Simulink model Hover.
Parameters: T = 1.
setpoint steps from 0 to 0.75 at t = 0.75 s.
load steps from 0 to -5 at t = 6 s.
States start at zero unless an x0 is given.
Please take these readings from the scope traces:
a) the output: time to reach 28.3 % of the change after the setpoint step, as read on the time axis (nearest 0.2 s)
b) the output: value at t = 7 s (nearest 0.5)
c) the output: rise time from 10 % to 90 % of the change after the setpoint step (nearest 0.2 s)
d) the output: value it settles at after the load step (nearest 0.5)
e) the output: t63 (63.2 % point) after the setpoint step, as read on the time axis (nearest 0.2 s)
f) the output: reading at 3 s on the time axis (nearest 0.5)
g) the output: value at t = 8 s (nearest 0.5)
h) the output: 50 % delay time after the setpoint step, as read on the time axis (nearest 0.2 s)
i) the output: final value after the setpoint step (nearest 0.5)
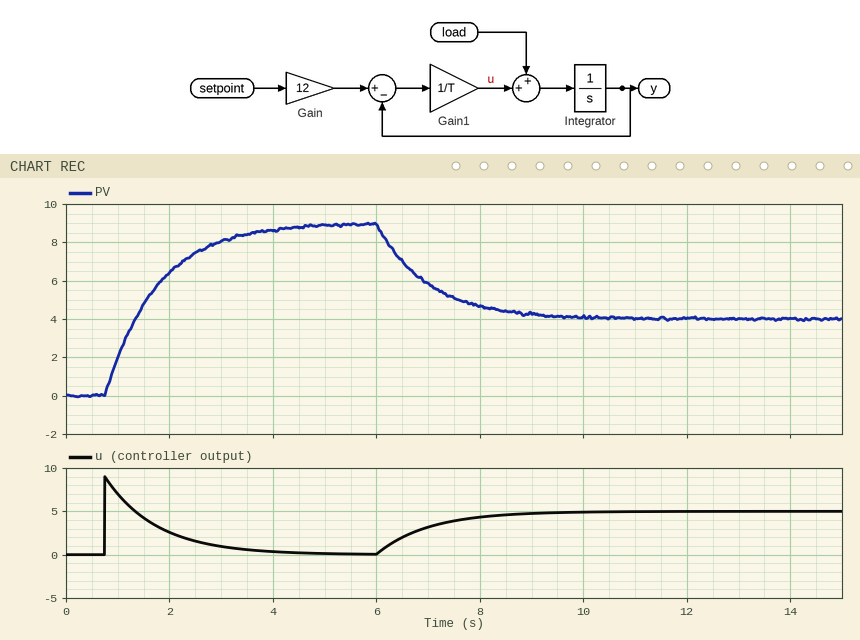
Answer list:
1.0 s
6.0
2.2 s
4.0
1.8 s
8.0
4.5
1.4 s
9.0
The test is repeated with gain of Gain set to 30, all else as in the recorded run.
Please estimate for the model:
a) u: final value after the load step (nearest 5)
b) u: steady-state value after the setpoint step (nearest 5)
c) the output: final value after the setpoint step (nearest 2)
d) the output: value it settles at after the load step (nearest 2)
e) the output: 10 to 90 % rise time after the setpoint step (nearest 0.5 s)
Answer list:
5
0
22
18
2.0 s
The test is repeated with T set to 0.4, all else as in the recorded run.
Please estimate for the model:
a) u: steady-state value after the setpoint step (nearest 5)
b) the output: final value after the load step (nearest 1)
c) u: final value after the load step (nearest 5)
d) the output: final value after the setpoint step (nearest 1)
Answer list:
0
7
5
9
